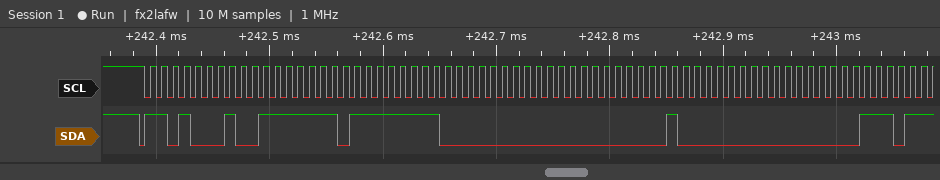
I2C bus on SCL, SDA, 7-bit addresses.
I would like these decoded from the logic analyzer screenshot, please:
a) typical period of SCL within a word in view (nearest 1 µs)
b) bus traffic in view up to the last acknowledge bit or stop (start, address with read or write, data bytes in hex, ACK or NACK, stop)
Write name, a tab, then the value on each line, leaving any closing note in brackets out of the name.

typical period of SCL within a word in view	10 µs
bus traffic in view up to the last acknowledge bit or stop	start, address 68 read ACK, 7F ACK, FF ACK, 00 ACK, 00 ACK, 40 ACK, 00 ACK
